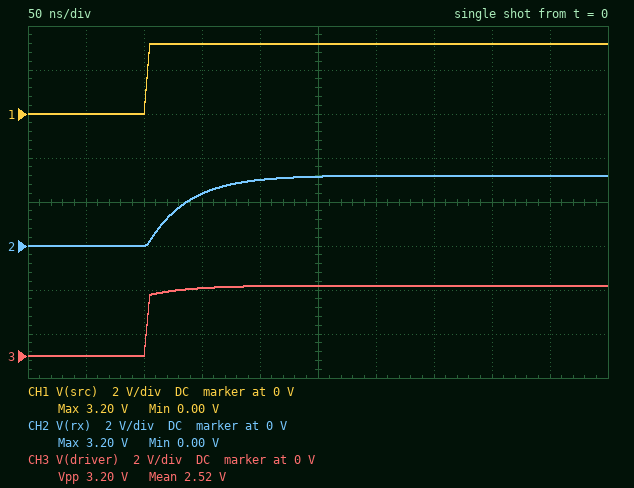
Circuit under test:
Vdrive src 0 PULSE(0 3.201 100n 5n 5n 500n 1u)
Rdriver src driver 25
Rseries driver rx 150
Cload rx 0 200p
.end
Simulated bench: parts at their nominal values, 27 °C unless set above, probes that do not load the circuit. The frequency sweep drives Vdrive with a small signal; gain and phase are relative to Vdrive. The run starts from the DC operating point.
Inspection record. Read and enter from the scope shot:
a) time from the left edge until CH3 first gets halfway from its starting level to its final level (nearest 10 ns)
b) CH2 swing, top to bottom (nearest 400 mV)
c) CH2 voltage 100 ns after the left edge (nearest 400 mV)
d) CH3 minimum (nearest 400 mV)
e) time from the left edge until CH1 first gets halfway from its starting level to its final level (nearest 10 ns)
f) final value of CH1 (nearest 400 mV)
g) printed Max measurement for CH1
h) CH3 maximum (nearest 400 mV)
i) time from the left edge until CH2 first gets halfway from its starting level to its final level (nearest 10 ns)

100 ns
3.2 V
0 V
0 V
100 ns
3.2 V
3.20 V
3.2 V
130 ns
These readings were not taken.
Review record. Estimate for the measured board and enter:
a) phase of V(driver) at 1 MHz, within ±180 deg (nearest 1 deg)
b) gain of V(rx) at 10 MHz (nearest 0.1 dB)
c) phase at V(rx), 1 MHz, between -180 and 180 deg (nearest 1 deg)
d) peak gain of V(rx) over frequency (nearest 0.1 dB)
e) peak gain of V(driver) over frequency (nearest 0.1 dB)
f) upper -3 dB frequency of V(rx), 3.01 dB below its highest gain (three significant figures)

-2 deg
-7.7 dB
-12 deg
0 dB
0 dB
4.55 MHz
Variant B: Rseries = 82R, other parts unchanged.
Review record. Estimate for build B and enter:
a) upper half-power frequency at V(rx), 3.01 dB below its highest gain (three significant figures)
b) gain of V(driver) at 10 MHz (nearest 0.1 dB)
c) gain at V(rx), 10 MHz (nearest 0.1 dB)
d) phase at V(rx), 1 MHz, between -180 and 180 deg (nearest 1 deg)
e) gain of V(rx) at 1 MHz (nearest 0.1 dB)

7.44 MHz
-1.3 dB
-4.5 dB
-8 deg
-0.1 dB
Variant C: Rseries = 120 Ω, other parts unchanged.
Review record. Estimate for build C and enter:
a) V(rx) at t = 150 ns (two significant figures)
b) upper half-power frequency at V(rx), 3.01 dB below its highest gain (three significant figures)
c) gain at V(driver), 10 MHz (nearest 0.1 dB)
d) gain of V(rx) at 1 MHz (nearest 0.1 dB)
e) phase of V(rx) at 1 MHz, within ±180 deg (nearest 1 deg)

2.6 V
5.49 MHz
-1.2 dB
-0.1 dB
-10 deg
